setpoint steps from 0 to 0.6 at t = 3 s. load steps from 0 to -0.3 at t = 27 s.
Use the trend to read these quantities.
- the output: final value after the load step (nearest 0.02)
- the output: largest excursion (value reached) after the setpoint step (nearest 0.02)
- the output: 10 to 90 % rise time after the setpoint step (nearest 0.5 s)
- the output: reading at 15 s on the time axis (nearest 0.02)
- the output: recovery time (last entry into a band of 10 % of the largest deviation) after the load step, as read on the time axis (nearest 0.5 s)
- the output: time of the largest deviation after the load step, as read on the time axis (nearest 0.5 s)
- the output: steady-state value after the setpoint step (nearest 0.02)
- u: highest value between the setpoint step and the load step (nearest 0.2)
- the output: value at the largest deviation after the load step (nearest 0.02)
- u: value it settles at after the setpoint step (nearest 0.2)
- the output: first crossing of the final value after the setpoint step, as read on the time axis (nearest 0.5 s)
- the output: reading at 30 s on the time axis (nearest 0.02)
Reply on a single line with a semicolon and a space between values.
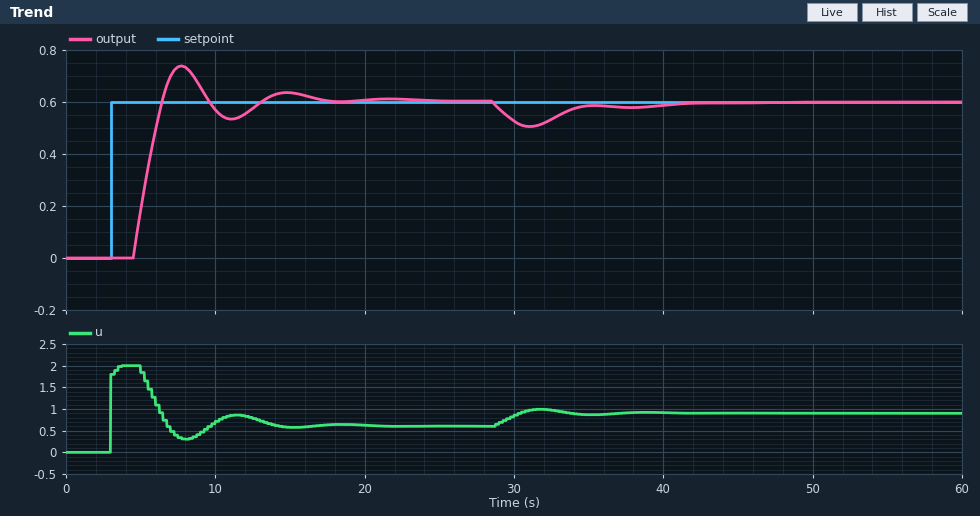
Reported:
0.60; 0.74; 1.5 s; 0.64; 40.5 s; 31.0 s; 0.60; 2.0; 0.50; 0.6; 6.5 s; 0.52
